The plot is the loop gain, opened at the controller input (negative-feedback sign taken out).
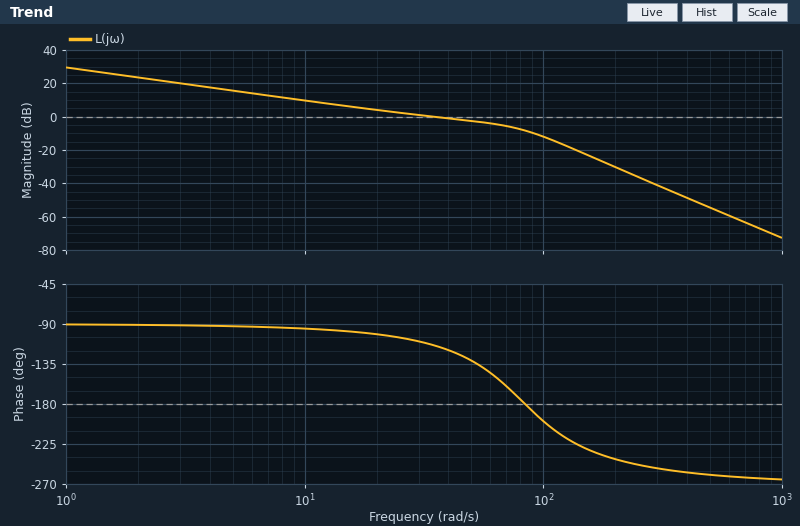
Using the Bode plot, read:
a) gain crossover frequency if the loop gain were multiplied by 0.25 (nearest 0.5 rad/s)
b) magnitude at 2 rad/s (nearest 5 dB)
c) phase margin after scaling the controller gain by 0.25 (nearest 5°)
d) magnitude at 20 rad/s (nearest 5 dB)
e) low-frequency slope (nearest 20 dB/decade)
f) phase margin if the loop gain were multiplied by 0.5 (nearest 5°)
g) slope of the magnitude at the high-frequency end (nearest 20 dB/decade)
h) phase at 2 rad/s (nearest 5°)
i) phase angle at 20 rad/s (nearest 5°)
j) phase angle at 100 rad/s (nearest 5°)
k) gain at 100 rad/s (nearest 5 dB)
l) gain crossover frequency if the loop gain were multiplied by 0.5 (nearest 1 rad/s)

7.5 rad/s
25 dB
85°
5 dB
-20 dB/decade
80°
-60 dB/decade
-90°
-100°
-200°
-10 dB
16 rad/s
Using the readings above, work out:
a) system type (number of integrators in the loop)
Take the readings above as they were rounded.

1
